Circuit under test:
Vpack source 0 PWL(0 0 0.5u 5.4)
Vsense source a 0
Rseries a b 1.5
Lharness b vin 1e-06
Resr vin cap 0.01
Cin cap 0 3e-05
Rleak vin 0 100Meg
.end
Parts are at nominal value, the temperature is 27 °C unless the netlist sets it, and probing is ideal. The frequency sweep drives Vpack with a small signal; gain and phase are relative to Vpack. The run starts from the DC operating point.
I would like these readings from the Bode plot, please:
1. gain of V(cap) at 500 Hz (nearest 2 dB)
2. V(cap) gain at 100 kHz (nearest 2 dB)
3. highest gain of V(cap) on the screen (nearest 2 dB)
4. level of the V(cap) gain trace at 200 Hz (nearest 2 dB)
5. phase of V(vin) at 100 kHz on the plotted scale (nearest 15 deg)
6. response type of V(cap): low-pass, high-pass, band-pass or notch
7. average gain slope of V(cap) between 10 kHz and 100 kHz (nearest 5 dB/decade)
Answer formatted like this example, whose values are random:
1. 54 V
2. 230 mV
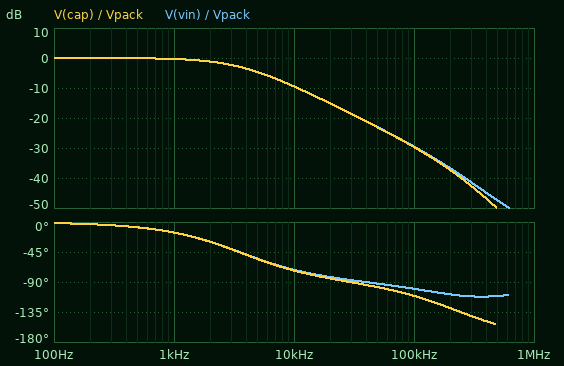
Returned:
1. 0 dB
2. -30 dB
3. 0 dB
4. 0 dB
5. -105 deg
6. low-pass
7. -20 dB/decade
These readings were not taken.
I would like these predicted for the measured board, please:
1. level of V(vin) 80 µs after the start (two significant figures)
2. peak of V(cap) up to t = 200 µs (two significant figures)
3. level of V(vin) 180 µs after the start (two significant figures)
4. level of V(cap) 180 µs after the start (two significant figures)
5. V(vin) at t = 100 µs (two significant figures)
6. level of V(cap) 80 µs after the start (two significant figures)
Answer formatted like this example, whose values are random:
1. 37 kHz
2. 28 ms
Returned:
1. 4.5 V
2. 5.3 V
3. 5.3 V
4. 5.3 V
5. 4.8 V
6. 4.5 V
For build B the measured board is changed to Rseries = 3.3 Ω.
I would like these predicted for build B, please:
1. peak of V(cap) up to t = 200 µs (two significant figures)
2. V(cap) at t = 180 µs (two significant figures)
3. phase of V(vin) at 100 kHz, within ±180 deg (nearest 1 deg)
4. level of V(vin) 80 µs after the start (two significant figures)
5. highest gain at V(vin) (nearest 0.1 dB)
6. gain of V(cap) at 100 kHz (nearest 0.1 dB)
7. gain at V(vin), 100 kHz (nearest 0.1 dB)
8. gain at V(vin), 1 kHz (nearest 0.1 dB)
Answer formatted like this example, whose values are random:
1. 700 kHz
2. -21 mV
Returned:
1. 4.7 V
2. 4.5 V
3. -89 deg
4. 3.0 V
5. 0 dB
6. -36.0 dB
7. -35.9 dB
8. -1.4 dB
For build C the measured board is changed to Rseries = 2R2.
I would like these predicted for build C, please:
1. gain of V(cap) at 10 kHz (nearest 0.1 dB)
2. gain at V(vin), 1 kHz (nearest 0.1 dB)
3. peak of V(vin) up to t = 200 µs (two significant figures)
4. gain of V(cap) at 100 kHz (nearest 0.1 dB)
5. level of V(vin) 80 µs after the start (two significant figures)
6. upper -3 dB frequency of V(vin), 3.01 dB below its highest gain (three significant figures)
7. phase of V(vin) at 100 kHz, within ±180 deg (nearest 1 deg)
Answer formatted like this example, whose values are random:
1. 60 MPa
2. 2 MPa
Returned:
1. -12.6 dB
2. -0.7 dB
3. 5.1 V
4. -32.7 dB
5. 3.8 V
6. 2.42 kHz
7. -94 deg
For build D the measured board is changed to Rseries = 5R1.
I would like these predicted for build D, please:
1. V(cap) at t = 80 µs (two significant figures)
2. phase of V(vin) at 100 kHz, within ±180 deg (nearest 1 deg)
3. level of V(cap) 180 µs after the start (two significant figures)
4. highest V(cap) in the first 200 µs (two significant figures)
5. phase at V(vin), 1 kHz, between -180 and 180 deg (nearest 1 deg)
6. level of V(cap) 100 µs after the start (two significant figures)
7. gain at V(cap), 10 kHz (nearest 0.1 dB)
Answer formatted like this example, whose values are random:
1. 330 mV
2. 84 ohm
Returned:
1. 2.2 V
2. -86 deg
3. 3.7 V
4. 3.9 V
5. -44 deg
6. 2.6 V
7. -19.7 dB
